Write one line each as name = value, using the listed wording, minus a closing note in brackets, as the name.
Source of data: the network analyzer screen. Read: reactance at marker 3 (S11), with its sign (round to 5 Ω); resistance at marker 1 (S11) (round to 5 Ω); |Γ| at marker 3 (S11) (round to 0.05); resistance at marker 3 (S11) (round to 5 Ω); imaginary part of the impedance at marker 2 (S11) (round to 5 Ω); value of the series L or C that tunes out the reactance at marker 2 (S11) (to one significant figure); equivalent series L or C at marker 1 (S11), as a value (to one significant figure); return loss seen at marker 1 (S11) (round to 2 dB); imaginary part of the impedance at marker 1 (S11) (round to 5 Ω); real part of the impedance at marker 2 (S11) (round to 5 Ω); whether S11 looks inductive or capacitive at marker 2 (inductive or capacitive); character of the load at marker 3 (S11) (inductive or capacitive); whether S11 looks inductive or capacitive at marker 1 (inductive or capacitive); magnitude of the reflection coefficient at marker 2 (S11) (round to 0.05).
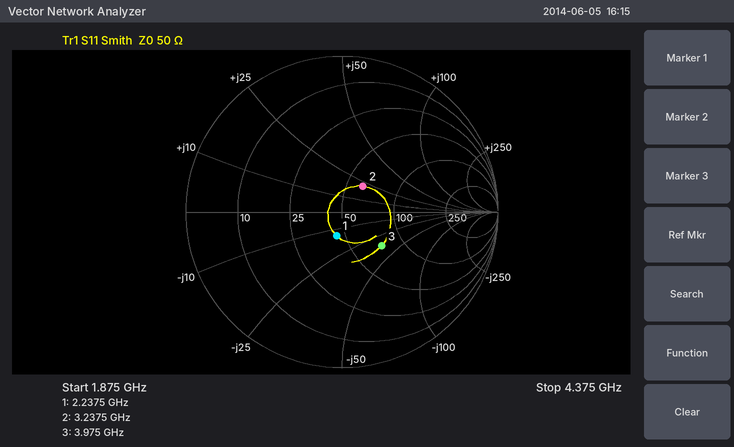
reactance at marker 3 (S11), with its sign = -35 Ω
resistance at marker 1 (S11) = 45 Ω
|Γ| at marker 3 (S11) = 0.35
resistance at marker 3 (S11) = 75 Ω
imaginary part of the impedance at marker 2 (S11) = +20 Ω
value of the series L or C that tunes out the reactance at marker 2 (S11) = 2 pF
equivalent series L or C at marker 1 (S11), as a value = 5 pF
return loss seen at marker 1 (S11) = 16 dB
imaginary part of the impedance at marker 1 (S11) = -15 Ω
real part of the impedance at marker 2 (S11) = 60 Ω
whether S11 looks inductive or capacitive at marker 2 = inductive
character of the load at marker 3 (S11) = capacitive
whether S11 looks inductive or capacitive at marker 1 = capacitive
magnitude of the reflection coefficient at marker 2 (S11) = 0.20
